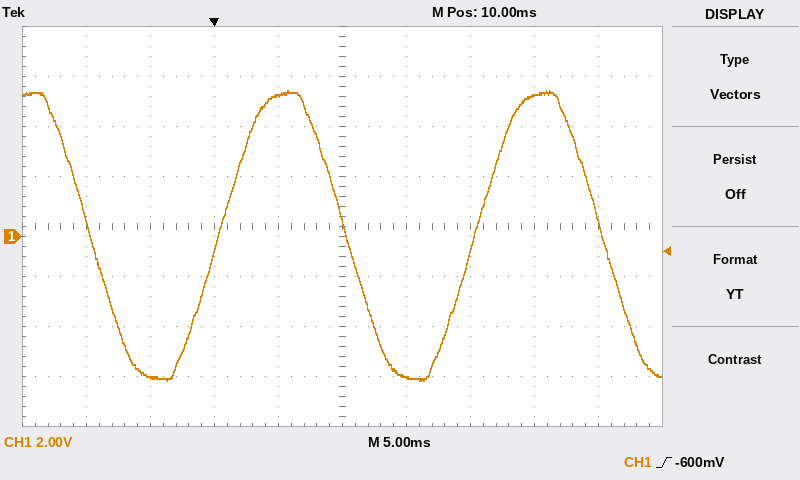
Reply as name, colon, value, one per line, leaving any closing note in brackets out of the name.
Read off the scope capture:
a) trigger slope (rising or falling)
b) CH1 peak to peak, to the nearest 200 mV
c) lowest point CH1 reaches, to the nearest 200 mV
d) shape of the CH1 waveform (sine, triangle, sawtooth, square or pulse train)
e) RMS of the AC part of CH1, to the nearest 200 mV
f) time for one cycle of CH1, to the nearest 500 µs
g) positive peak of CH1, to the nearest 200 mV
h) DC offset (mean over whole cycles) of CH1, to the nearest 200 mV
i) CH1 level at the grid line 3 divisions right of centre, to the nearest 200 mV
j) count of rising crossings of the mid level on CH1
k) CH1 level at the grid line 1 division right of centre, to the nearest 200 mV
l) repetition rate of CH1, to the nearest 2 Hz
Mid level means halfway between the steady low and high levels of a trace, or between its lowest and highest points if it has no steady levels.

trigger slope: rising
CH1 peak to peak, to the nearest 200 mV: 11.6 V
lowest point CH1 reaches, to the nearest 200 mV: -5.8 V
shape of the CH1 waveform: sine
RMS of the AC part of CH1, to the nearest 200 mV: 4.2 V
time for one cycle of CH1, to the nearest 500 µs: 20.0 ms
positive peak of CH1, to the nearest 200 mV: 5.8 V
DC offset (mean over whole cycles) of CH1, to the nearest 200 mV: 0.0 V
CH1 level at the grid line 3 divisions right of centre, to the nearest 200 mV: 5.6 V
count of rising crossings of the mid level on CH1: 2
CH1 level at the grid line 1 division right of centre, to the nearest 200 mV: -5.6 V
repetition rate of CH1, to the nearest 2 Hz: 50 Hz
